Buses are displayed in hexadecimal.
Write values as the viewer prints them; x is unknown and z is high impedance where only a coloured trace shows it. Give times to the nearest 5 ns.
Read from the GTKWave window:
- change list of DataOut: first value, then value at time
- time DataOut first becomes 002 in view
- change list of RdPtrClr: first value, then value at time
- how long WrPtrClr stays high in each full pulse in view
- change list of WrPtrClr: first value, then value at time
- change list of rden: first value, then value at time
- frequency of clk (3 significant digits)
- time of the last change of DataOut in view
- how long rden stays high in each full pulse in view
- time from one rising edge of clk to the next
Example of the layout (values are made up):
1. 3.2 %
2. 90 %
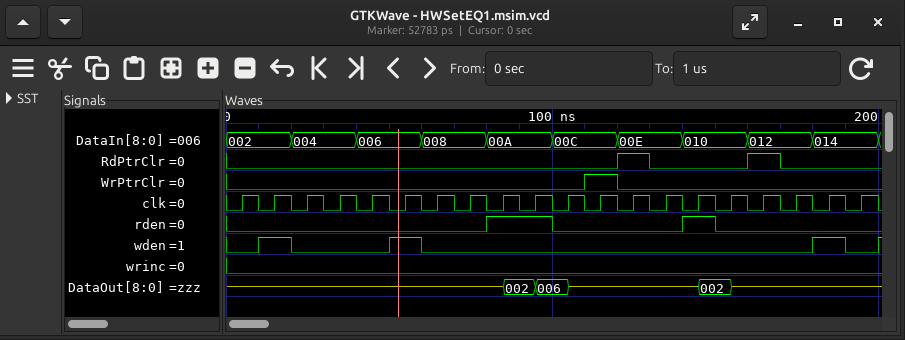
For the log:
1. z, 002 at 85 ns, 006 at 95 ns, z at 105 ns, 002 at 145 ns, z at 155 ns
2. 85 ns
3. 0, 1 at 120 ns, 0 at 130 ns, 1 at 160 ns, 0 at 170 ns
4. 10 ns
5. 0, 1 at 110 ns, 0 at 120 ns
6. 0, 1 at 80 ns, 0 at 100 ns, 1 at 140 ns, 0 at 150 ns
7. 100 MHz
8. 155 ns
9. 20 ns, 10 ns
10. 10 ns
